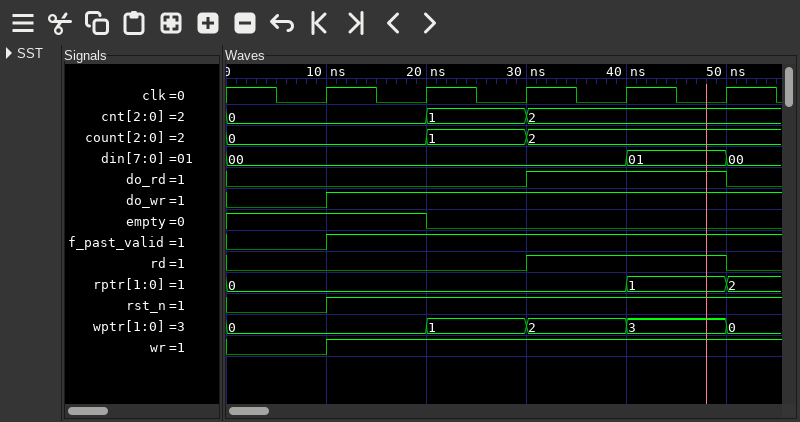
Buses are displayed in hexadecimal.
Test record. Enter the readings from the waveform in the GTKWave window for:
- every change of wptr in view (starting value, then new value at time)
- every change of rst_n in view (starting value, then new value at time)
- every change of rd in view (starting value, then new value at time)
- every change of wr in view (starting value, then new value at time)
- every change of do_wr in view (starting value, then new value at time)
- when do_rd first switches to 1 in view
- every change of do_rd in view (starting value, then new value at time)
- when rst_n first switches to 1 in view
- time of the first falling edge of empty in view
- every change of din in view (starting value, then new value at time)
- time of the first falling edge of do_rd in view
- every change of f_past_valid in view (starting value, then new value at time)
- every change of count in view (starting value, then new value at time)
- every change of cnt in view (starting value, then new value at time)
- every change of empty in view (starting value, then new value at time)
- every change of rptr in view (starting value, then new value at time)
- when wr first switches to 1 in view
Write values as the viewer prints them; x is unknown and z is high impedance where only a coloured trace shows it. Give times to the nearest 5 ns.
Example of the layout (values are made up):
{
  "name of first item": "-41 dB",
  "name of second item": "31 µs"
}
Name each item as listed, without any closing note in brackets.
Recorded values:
{
  "every change of wptr in view": "0, 1 at 20 ns, 2 at 30 ns, 3 at 40 ns, 0 at 50 ns",
  "every change of rst_n in view": "0, 1 at 10 ns",
  "every change of rd in view": "0, 1 at 30 ns, 0 at 50 ns",
  "every change of wr in view": "0, 1 at 10 ns",
  "every change of do_wr in view": "0, 1 at 10 ns",
  "when do_rd first switches to 1 in view": "30 ns",
  "every change of do_rd in view": "0, 1 at 30 ns, 0 at 50 ns",
  "when rst_n first switches to 1 in view": "10 ns",
  "time of the first falling edge of empty in view": "20 ns",
  "every change of din in view": "00, 01 at 40 ns, 00 at 50 ns",
  "time of the first falling edge of do_rd in view": "50 ns",
  "every change of f_past_valid in view": "0, 1 at 10 ns",
  "every change of count in view": "0, 1 at 20 ns, 2 at 30 ns",
  "every change of cnt in view": "0, 1 at 20 ns, 2 at 30 ns",
  "every change of empty in view": "1, 0 at 20 ns",
  "every change of rptr in view": "0, 1 at 40 ns, 2 at 50 ns",
  "when wr first switches to 1 in view": "10 ns"
}
